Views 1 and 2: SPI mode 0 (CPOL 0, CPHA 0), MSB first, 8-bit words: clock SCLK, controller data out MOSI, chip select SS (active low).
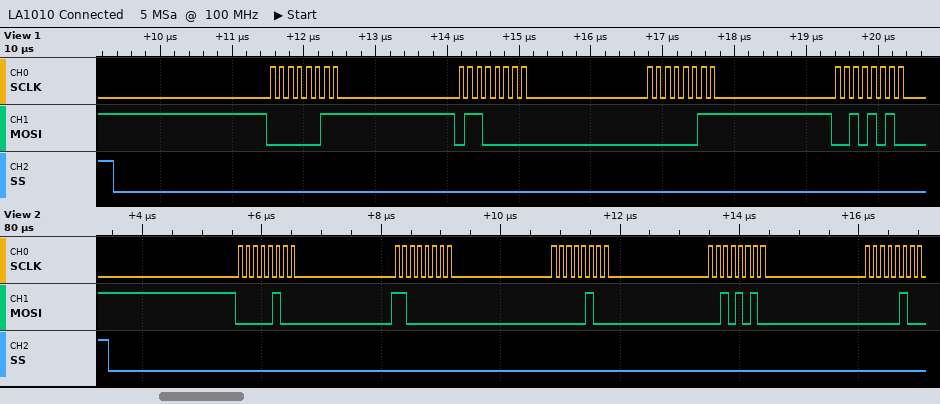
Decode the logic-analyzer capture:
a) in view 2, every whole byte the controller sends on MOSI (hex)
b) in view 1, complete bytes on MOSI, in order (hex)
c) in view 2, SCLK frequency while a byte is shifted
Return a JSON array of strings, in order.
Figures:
["04 C0 04 2A 04", "03 60 03 2A", "8 MHz"]
